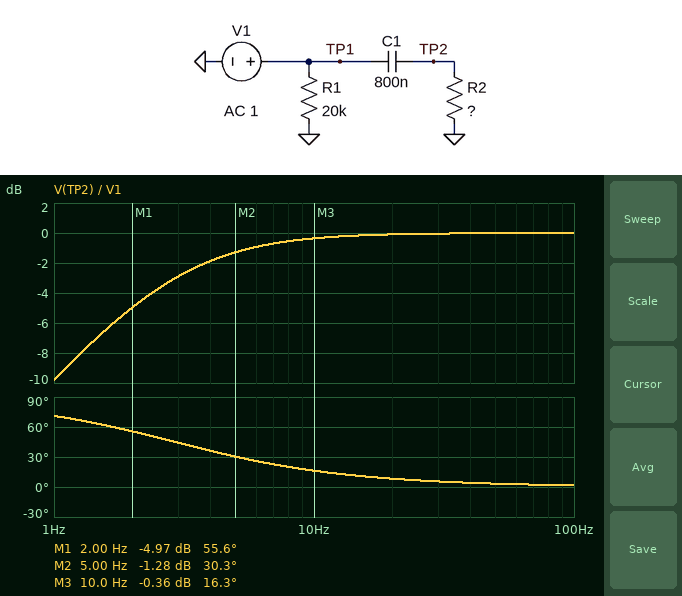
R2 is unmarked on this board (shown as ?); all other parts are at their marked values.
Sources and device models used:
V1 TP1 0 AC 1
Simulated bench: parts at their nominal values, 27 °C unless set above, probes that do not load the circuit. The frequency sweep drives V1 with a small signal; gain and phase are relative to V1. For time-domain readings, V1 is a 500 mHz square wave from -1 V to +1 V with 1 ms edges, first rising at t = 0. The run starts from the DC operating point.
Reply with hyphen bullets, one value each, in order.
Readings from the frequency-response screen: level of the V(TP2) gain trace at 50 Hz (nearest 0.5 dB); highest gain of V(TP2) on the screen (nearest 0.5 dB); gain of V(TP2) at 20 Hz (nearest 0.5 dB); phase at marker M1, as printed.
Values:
- 0 dB
- 0 dB
- 0 dB
- 55.6 deg
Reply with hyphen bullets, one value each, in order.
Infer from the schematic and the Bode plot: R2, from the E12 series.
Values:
- 68 kΩ
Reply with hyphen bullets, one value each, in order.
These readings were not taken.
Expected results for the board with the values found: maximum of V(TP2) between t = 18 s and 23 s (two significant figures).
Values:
- 2.0 V
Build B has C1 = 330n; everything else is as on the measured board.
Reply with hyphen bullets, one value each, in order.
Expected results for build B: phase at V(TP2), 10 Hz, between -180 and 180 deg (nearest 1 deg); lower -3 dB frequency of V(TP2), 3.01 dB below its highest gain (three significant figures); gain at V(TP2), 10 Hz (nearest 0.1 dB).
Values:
- 35 deg
- 7.09 Hz
- -1.8 dB
